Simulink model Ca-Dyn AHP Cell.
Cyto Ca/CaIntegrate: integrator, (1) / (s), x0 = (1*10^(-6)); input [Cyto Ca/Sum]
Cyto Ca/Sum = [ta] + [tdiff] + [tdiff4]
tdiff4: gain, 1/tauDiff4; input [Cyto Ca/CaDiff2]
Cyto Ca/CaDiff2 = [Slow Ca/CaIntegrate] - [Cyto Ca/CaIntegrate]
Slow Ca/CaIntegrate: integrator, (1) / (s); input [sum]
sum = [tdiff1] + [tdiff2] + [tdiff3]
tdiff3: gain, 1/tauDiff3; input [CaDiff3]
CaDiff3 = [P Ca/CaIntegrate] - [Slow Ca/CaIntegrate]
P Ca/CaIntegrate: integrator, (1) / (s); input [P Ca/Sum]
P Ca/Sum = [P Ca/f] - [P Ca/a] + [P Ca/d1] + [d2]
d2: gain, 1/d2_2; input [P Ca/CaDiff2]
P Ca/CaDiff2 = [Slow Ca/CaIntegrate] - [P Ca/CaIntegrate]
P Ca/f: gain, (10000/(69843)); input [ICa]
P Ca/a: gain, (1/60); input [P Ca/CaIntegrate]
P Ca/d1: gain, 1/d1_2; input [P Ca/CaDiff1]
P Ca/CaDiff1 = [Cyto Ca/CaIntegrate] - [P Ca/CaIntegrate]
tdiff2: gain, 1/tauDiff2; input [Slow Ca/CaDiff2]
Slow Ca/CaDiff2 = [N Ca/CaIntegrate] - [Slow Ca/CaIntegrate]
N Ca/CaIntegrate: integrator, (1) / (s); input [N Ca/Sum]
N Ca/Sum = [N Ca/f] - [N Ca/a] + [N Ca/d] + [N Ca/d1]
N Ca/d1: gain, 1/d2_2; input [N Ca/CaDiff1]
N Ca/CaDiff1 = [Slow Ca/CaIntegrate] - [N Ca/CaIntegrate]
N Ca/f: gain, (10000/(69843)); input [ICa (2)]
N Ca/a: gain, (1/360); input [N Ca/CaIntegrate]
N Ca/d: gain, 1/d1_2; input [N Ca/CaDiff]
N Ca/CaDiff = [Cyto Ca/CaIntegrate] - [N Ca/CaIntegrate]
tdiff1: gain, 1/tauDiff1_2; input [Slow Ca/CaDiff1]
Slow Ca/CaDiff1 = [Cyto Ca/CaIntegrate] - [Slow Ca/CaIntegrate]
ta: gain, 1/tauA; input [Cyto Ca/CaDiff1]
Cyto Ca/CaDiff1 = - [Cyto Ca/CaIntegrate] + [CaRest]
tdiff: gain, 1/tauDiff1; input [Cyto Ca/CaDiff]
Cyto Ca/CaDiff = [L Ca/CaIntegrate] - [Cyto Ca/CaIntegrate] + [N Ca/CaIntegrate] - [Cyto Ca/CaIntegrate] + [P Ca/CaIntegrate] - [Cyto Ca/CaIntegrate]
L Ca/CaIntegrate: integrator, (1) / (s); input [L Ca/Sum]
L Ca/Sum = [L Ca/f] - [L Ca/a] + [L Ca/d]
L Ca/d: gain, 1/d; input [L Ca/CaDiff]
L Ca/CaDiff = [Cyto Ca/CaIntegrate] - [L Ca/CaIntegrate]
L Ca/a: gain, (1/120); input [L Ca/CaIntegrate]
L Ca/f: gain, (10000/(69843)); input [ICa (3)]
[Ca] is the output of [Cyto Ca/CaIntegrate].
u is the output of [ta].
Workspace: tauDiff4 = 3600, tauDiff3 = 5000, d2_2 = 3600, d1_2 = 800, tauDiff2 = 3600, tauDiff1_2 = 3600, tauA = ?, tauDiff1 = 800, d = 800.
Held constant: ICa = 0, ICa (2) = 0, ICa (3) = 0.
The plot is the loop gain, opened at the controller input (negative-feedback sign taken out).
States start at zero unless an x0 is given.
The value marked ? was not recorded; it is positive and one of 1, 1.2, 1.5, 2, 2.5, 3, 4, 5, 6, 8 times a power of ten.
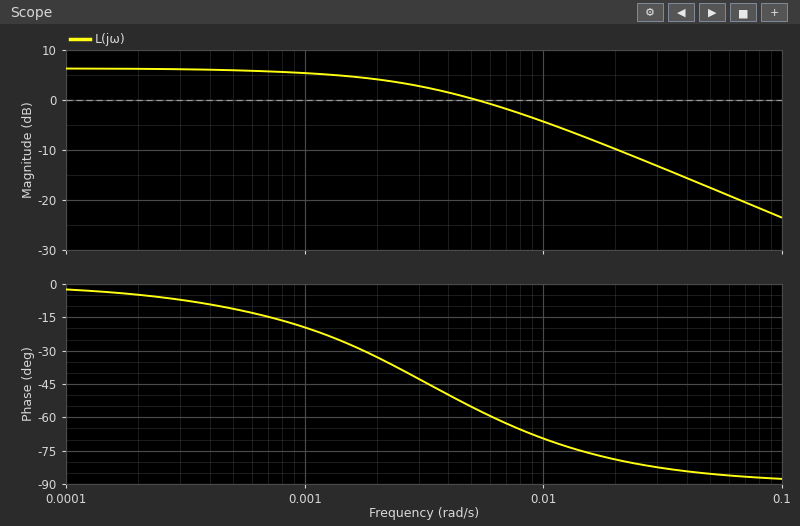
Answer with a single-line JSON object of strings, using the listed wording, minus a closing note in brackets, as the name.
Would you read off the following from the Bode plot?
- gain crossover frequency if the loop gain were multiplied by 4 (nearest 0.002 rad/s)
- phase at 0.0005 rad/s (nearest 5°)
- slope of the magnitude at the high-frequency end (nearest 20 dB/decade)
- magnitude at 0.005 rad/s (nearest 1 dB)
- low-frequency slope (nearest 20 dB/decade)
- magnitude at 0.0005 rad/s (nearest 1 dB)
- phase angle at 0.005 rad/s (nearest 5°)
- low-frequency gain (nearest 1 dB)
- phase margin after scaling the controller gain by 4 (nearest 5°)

{"gain crossover frequency if the loop gain were multiplied by 4": "0.026 rad/s", "phase at 0.0005 rad/s": "-10°", "slope of the magnitude at the high-frequency end": "-20 dB/decade", "magnitude at 0.005 rad/s": "0 dB", "low-frequency slope": "0 dB/decade", "magnitude at 0.0005 rad/s": "6 dB", "phase angle at 0.005 rad/s": "-55°", "low-frequency gain": "6 dB", "phase margin after scaling the controller gain by 4": "100°"}
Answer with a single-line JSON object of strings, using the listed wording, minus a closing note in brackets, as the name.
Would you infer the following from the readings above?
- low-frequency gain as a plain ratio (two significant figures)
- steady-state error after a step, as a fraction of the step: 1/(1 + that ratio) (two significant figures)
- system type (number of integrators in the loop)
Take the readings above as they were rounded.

{"low-frequency gain as a plain ratio": "2.0", "steady-state error after a step, as a fraction of the step: 1/(1 + that ratio)": "0.33", "system type": "0"}
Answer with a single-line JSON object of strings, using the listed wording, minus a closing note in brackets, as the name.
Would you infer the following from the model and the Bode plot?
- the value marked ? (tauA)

{"the value marked ?": "150"}
